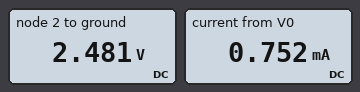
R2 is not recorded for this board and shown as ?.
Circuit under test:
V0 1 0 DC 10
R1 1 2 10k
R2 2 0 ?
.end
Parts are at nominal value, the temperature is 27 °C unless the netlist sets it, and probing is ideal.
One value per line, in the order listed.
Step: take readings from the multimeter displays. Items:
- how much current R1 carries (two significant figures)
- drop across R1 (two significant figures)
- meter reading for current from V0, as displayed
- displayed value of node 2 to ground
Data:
750 µA
7.5 V
0.752 mA
2.481 V
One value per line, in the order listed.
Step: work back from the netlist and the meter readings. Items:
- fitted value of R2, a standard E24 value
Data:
3.3 kΩ
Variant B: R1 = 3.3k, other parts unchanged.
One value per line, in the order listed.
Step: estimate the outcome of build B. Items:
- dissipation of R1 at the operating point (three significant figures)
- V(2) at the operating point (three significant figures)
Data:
7.58 mW
5.00 V
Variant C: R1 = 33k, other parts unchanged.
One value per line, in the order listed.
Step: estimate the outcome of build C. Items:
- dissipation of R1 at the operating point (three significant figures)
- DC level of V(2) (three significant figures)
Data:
2.50 mW
909 mV
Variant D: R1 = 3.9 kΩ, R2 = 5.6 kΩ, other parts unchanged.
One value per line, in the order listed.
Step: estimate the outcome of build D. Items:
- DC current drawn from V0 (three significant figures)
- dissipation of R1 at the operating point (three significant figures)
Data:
1.05 mA
4.32 mW
